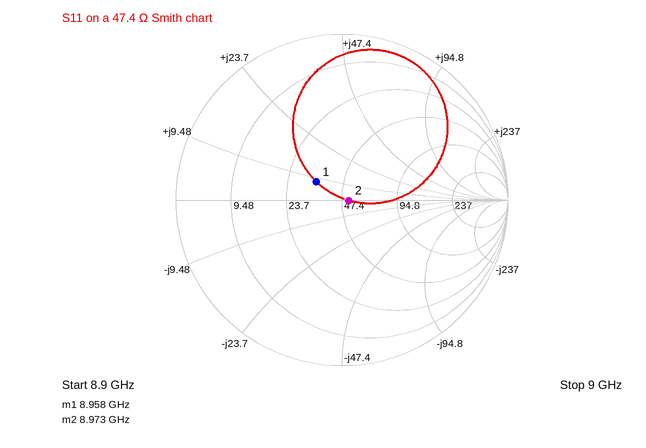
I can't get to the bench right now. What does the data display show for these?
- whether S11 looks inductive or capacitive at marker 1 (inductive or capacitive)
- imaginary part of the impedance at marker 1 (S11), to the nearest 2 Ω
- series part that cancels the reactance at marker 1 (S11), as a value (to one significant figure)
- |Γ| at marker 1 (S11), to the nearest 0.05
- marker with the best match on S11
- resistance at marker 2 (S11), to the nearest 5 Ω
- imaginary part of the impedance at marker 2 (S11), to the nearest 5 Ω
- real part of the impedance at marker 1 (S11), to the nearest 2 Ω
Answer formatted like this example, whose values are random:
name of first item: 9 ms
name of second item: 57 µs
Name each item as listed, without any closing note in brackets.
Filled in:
whether S11 looks inductive or capacitive at marker 1: inductive
imaginary part of the impedance at marker 1 (S11), to the nearest 2 Ω: +8 Ω
series part that cancels the reactance at marker 1 (S11), as a value: 2 pF
|Γ| at marker 1 (S11), to the nearest 0.05: 0.20
marker with the best match on S11: marker 2
resistance at marker 2 (S11), to the nearest 5 Ω: 50 Ω
imaginary part of the impedance at marker 2 (S11), to the nearest 5 Ω: 0 Ω
real part of the impedance at marker 1 (S11), to the nearest 2 Ω: 34 Ω
